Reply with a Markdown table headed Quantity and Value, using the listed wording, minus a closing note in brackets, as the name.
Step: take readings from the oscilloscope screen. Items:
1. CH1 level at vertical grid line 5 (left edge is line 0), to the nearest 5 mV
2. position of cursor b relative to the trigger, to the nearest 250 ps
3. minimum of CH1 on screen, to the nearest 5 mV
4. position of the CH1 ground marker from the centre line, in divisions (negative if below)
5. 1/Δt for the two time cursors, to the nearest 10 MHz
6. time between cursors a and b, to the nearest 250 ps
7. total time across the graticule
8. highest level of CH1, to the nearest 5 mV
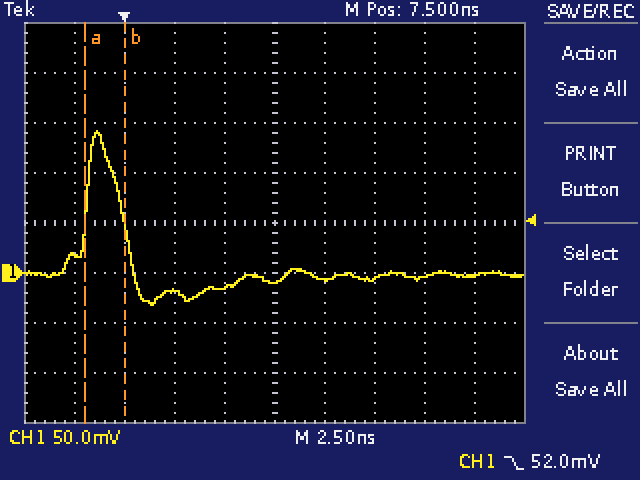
| Quantity | Value |
|---|---|
| CH1 level at vertical grid line 5 (left edge is line 0), to the nearest 5 mV | -10 mV |
| position of cursor b relative to the trigger, to the nearest 250 ps | 0.00 ns |
| minimum of CH1 on screen, to the nearest 5 mV | -30 mV |
| position of the CH1 ground marker from the centre line, in divisions | -1.0 div |
| 1/Δt for the two time cursors, to the nearest 10 MHz | 500 MHz |
| time between cursors a and b, to the nearest 250 ps | 2.00 ns |
| total time across the graticule | 25 ns |
| highest level of CH1, to the nearest 5 mV | 140 mV |
